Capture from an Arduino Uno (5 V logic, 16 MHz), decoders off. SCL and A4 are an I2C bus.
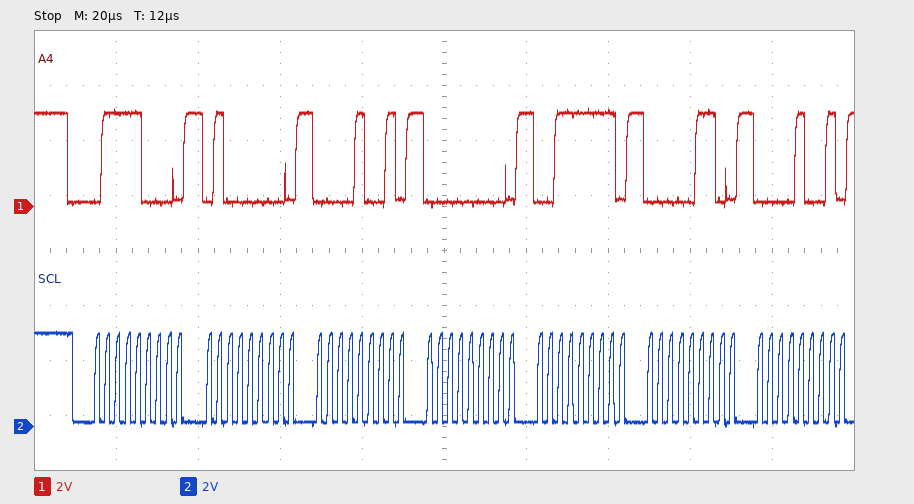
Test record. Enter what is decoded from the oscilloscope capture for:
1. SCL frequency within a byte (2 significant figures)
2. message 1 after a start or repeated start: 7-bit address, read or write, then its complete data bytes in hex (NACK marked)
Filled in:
400 kHz
0x3C write: 40 09 00 3F 06 09
